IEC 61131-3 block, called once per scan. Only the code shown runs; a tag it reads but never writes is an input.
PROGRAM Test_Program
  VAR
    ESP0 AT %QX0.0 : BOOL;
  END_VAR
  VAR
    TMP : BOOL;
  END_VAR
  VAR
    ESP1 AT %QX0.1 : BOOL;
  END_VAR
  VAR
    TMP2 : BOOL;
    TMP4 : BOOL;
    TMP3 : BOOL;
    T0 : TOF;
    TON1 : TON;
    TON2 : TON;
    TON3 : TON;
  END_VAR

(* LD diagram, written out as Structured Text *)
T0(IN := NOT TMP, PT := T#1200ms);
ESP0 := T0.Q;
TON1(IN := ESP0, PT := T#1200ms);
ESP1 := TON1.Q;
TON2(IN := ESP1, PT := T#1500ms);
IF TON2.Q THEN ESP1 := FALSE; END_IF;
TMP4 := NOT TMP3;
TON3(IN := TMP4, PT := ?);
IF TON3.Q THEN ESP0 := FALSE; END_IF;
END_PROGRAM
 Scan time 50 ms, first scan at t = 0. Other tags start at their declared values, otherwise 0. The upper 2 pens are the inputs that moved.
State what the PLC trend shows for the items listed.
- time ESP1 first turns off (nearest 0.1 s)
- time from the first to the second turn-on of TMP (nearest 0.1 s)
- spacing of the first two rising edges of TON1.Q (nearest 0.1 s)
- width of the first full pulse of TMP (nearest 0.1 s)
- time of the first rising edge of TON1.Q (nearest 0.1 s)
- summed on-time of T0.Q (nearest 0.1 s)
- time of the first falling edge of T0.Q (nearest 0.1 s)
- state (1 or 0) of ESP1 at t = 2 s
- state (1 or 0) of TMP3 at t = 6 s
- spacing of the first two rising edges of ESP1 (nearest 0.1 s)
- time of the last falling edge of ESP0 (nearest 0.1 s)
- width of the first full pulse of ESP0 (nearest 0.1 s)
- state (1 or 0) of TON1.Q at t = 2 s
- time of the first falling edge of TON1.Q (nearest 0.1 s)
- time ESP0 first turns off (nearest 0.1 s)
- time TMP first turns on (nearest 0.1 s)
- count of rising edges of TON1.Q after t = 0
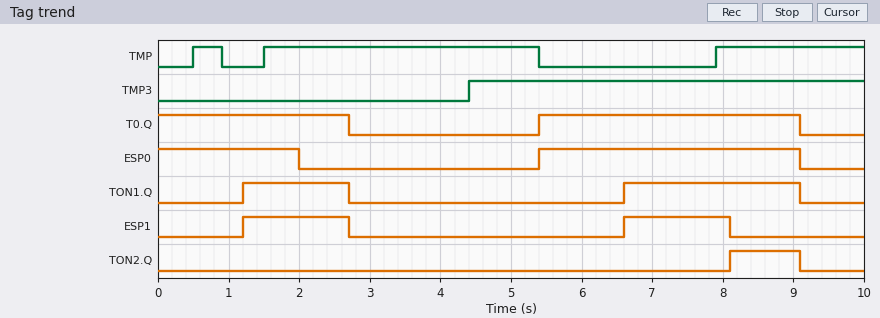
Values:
2.7 s
1.0 s
5.4 s
0.4 s
1.2 s
6.4 s
2.7 s
1
1
5.4 s
9.1 s
3.7 s
1
2.7 s
2.0 s
0.5 s
2
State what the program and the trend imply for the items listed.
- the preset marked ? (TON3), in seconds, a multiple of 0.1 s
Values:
2.0 s
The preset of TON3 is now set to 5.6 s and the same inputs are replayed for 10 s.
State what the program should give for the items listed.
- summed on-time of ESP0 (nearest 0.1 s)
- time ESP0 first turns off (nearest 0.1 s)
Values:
6.4 s
2.7 s
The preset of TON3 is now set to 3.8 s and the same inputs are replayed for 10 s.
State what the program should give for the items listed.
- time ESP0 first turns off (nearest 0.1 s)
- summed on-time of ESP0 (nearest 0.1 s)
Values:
2.7 s
6.4 s
